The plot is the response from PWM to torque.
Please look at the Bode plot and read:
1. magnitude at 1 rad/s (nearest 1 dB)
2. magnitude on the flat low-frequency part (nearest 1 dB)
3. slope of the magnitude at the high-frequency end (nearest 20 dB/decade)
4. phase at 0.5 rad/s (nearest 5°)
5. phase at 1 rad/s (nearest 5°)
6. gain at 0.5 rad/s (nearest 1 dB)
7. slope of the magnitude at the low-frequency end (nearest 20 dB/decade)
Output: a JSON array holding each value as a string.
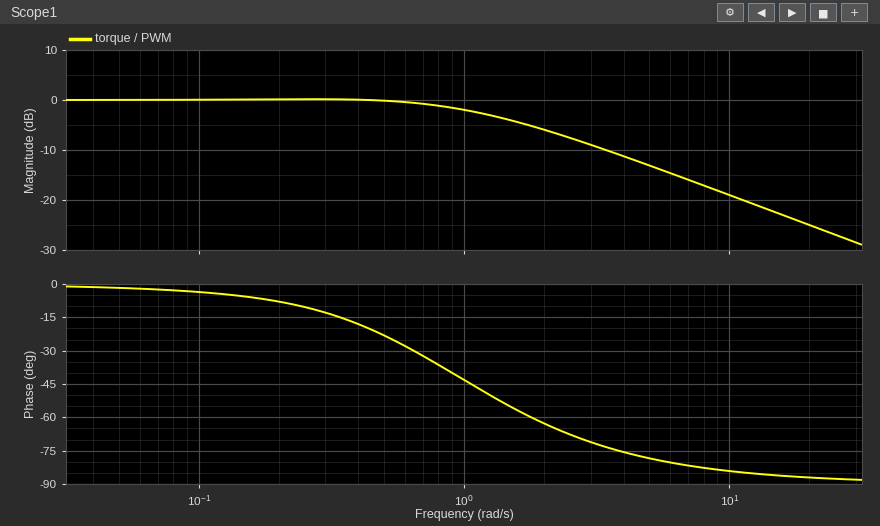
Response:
["-2 dB", "0 dB", "-20 dB/decade", "-25°", "-45°", "0 dB", "0 dB/decade"]
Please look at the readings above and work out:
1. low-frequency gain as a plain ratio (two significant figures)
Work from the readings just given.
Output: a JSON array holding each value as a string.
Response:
["1.0"]
